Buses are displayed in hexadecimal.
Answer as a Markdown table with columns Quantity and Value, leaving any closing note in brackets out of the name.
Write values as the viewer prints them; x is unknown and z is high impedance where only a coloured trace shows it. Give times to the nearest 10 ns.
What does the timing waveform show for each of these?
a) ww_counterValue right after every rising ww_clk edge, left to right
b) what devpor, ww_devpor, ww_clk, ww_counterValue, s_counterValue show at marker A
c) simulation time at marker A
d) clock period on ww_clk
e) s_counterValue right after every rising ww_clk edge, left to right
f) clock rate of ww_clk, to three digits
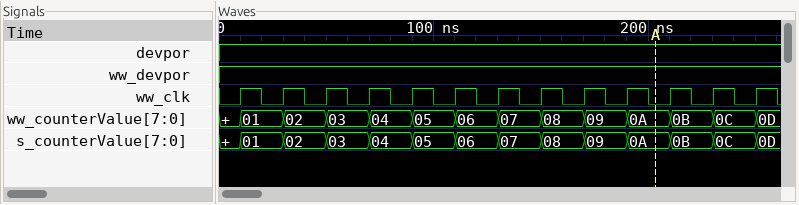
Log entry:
| Quantity | Value |
|---|---|
| ww_counterValue right after every rising ww_clk edge, left to right | 01, 02, 03, 04, 05, 06, 07, 08, 09, 0A, 0B, 0C, 0D |
| what devpor, ww_devpor, ww_clk, ww_counterValue, s_counterValue show at marker A | devpor=1, ww_devpor=1, ww_clk=0, ww_counterValue=0A, s_counterValue=0A |
| simulation time at marker A | 200 ns |
| clock period on ww_clk | 20 ns |
| s_counterValue right after every rising ww_clk edge, left to right | 01, 02, 03, 04, 05, 06, 07, 08, 09, 0A, 0B, 0C, 0D |
| clock rate of ww_clk, to three digits | 50.0 MHz |
